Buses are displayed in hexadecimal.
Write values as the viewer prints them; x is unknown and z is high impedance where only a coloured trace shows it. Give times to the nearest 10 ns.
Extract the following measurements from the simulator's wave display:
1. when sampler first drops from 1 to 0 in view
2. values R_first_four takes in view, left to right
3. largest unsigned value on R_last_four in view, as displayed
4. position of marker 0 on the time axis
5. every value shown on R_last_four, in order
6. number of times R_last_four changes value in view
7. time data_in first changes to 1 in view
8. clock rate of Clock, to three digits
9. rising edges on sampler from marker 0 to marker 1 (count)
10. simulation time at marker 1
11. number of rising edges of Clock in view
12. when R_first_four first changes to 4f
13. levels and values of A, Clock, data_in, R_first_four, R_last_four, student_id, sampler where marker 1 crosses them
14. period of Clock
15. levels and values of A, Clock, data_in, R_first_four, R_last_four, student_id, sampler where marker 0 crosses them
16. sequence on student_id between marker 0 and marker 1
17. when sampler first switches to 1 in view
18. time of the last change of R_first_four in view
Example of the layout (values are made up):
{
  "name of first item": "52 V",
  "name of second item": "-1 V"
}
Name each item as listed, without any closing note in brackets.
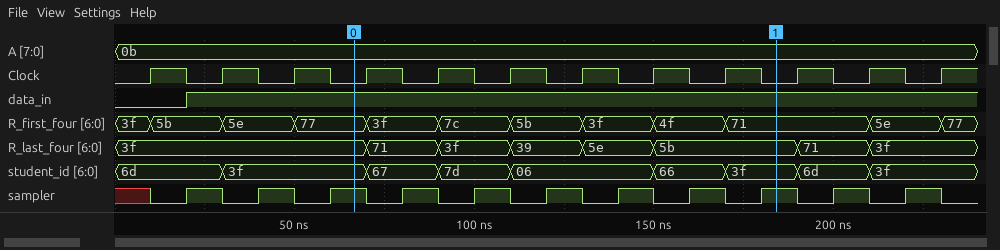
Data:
{
  "when sampler first drops from 1 to 0 in view": "30 ns",
  "values R_first_four takes in view, left to right": "3f, 5b, 5e, 77, 3f, 7c, 5b, 3f, 4f, 71, 5e, 77",
  "largest unsigned value on R_last_four in view, as displayed": "71",
  "position of marker 0 on the time axis": "70 ns",
  "every value shown on R_last_four, in order": "3f, 71, 3f, 39, 5e, 5b, 71, 3f",
  "number of times R_last_four changes value in view": "7",
  "time data_in first changes to 1 in view": "20 ns",
  "clock rate of Clock, to three digits": "50.0 MHz",
  "rising edges on sampler from marker 0 to marker 1": "6",
  "simulation time at marker 1": "180 ns",
  "number of rising edges of Clock in view": "12",
  "when R_first_four first changes to 4f": "150 ns",
  "levels and values of A, Clock, data_in, R_first_four, R_last_four, student_id, sampler where marker 1 crosses them": "A=0b, Clock=0, data_in=1, R_first_four=71, R_last_four=5b, student_id=3f, sampler=1",
  "period of Clock": "20 ns",
  "levels and values of A, Clock, data_in, R_first_four, R_last_four, student_id, sampler where marker 0 crosses them": "A=0b, Clock=0, data_in=1, R_first_four=77, R_last_four=3f, student_id=3f, sampler=1",
  "sequence on student_id between marker 0 and marker 1": "3f, 67, 7d, 06, 66, 3f",
  "when sampler first switches to 1 in view": "20 ns",
  "time of the last change of R_first_four in view": "230 ns"
}
